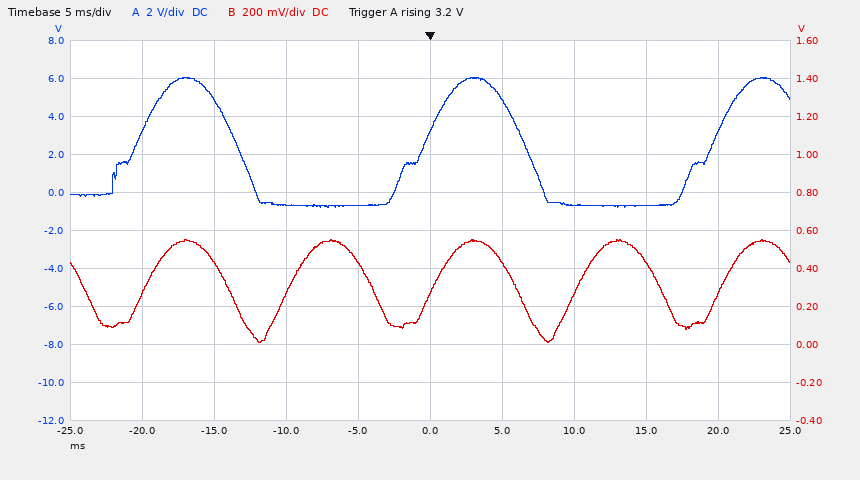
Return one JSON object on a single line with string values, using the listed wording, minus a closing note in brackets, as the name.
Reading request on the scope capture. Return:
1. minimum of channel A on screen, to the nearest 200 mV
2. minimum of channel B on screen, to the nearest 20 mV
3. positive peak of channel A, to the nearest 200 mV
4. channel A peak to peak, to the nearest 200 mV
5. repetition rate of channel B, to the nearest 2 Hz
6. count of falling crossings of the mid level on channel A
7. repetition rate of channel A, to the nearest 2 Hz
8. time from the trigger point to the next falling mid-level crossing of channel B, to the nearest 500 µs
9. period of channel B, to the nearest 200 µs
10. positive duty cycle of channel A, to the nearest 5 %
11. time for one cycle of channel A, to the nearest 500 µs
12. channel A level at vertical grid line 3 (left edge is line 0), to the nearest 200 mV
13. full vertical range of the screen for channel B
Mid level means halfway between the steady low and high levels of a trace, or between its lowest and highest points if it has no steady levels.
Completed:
{"minimum of channel A on screen, to the nearest 200 mV": "-800 mV", "minimum of channel B on screen, to the nearest 20 mV": "20 mV", "positive peak of channel A, to the nearest 200 mV": "6.0 V", "channel A peak to peak, to the nearest 200 mV": "6.8 V", "repetition rate of channel B, to the nearest 2 Hz": "100 Hz", "count of falling crossings of the mid level on channel A": "2", "repetition rate of channel A, to the nearest 2 Hz": "50 Hz", "time from the trigger point to the next falling mid-level crossing of channel B, to the nearest 500 µs": "6.0 ms", "period of channel B, to the nearest 200 µs": "10.0 ms", "positive duty cycle of channel A, to the nearest 5 %": "35 %", "time for one cycle of channel A, to the nearest 500 µs": "20.0 ms", "channel A level at vertical grid line 3 (left edge is line 0), to the nearest 200 mV": "-600 mV", "full vertical range of the screen for channel B": "2 V"}
